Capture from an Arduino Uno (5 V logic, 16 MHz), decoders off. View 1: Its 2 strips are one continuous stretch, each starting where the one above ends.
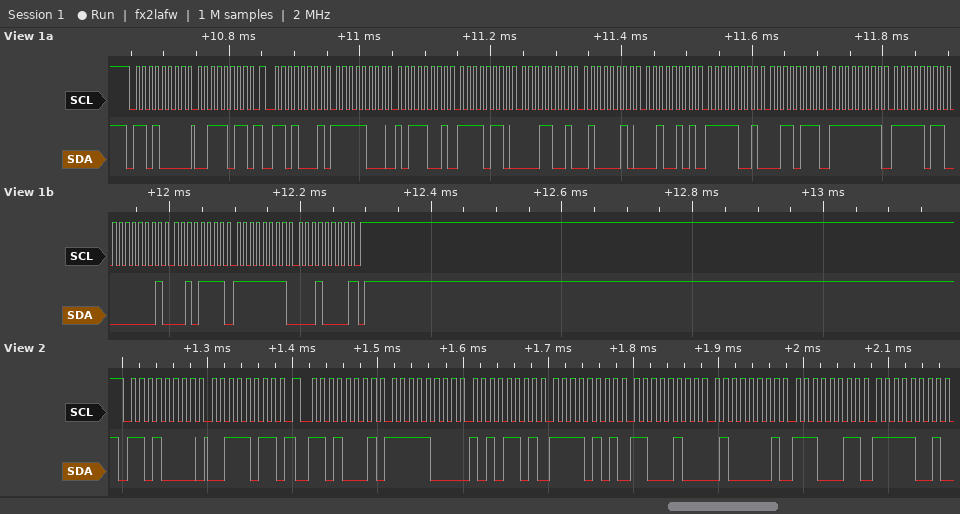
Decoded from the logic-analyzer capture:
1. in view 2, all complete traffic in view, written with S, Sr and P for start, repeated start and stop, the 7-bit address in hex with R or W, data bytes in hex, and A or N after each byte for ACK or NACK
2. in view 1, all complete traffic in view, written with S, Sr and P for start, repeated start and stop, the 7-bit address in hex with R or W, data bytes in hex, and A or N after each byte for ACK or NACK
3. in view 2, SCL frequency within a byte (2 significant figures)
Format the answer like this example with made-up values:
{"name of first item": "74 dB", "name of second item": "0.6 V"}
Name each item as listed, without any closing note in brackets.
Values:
{"in view 2, all complete traffic in view, written with S, Sr and P for start, repeated start and stop, the 7-bit address in hex with R or W, data bytes in hex, and A or N after each byte for ACK or NACK": "S 68W A 3B A Sr 68R A F8 A AD A F5 A C4 A 41 A E3 A F9 A", "in view 1, all complete traffic in view, written with S, Sr and P for start, repeated start and stop, the 7-bit address in hex with R or W, data bytes in hex, and A or N after each byte for ACK or NACK": "S 68W A 3B A Sr 68R A F8 A B9 A F6 A 19 A 42 A 25 A F9 A 37 A FF A FB A 01 A 2F A FF A 10 N P", "in view 2, SCL frequency within a byte": "100 kHz"}
